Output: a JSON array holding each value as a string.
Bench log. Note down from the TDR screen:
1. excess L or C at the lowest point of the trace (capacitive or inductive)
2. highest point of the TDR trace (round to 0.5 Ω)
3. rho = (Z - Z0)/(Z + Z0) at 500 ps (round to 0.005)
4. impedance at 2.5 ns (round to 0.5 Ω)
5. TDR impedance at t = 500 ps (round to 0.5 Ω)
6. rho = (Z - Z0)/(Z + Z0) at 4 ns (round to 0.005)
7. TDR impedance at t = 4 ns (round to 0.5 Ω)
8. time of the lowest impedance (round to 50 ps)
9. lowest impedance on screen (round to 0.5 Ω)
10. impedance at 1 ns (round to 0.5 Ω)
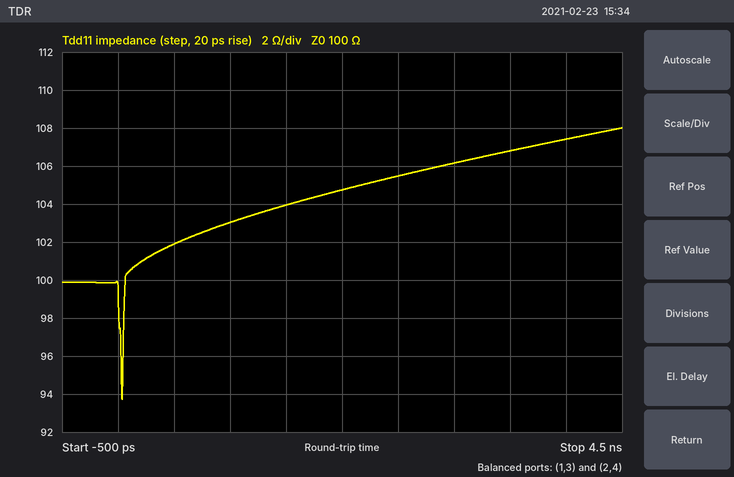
["capacitive", "108.0 Ω", "+0.010", "105.5 Ω", "102.0 Ω", "+0.035", "107.5 Ω", "50 ps", "93.5 Ω", "103.0 Ω"]
